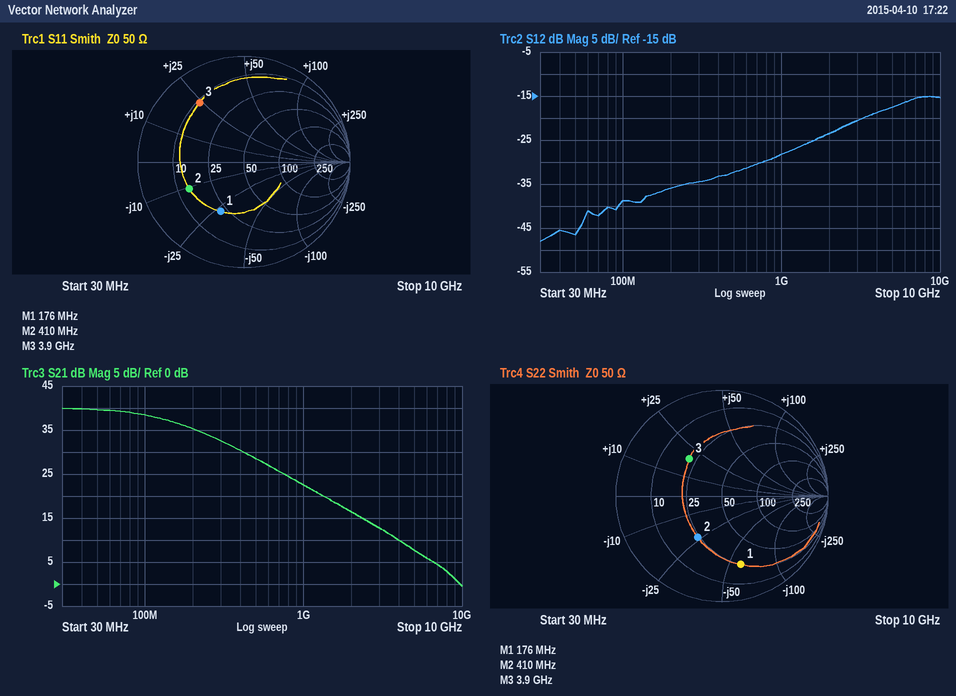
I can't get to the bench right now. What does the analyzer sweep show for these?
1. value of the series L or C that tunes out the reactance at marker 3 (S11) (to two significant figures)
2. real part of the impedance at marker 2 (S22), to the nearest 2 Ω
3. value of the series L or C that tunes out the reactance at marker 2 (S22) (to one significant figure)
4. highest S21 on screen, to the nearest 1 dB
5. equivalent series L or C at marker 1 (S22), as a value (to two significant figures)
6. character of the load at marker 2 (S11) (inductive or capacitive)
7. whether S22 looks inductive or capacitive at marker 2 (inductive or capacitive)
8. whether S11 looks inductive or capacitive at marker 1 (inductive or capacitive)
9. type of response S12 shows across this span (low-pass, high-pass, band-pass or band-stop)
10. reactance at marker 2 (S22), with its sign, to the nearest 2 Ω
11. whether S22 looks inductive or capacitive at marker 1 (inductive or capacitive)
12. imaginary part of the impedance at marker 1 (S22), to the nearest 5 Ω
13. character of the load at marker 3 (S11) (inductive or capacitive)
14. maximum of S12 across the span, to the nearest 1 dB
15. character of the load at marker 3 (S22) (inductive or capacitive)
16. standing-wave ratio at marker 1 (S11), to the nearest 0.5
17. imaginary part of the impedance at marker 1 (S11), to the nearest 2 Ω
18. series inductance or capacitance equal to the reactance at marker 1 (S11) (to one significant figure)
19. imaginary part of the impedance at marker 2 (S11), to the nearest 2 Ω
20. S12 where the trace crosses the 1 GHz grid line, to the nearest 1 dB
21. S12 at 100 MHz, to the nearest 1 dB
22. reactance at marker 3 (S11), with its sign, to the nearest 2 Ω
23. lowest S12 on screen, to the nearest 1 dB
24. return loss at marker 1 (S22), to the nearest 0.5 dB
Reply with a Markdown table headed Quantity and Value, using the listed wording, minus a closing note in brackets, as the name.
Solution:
| Quantity | Value |
|---|---|
| value of the series L or C that tunes out the reactance at marker 3 (S11) | 1.7 pF |
| real part of the impedance at marker 2 (S22), to the nearest 2 Ω | 24 Ω |
| value of the series L or C that tunes out the reactance at marker 2 (S22) | 9 nH |
| highest S21 on screen, to the nearest 1 dB | 40 dB |
| equivalent series L or C at marker 1 (S22), as a value | 15 pF |
| character of the load at marker 2 (S11) | capacitive |
| whether S22 looks inductive or capacitive at marker 2 | capacitive |
| whether S11 looks inductive or capacitive at marker 1 | capacitive |
| type of response S12 shows across this span | high-pass |
| reactance at marker 2 (S22), with its sign, to the nearest 2 Ω | -24 Ω |
| whether S22 looks inductive or capacitive at marker 1 | capacitive |
| imaginary part of the impedance at marker 1 (S22), to the nearest 5 Ω | -60 Ω |
| character of the load at marker 3 (S11) | inductive |
| maximum of S12 across the span, to the nearest 1 dB | -15 dB |
| character of the load at marker 3 (S22) | inductive |
| standing-wave ratio at marker 1 (S11), to the nearest 0.5 | 3.0 |
| imaginary part of the impedance at marker 1 (S11), to the nearest 2 Ω | -28 Ω |
| series inductance or capacitance equal to the reactance at marker 1 (S11) | 30 pF |
| imaginary part of the impedance at marker 2 (S11), to the nearest 2 Ω | -10 Ω |
| S12 where the trace crosses the 1 GHz grid line, to the nearest 1 dB | -28 dB |
| S12 at 100 MHz, to the nearest 1 dB | -39 dB |
| reactance at marker 3 (S11), with its sign, to the nearest 2 Ω | +24 Ω |
| lowest S12 on screen, to the nearest 1 dB | -48 dB |
| return loss at marker 1 (S22), to the nearest 0.5 dB | 3.5 dB |
